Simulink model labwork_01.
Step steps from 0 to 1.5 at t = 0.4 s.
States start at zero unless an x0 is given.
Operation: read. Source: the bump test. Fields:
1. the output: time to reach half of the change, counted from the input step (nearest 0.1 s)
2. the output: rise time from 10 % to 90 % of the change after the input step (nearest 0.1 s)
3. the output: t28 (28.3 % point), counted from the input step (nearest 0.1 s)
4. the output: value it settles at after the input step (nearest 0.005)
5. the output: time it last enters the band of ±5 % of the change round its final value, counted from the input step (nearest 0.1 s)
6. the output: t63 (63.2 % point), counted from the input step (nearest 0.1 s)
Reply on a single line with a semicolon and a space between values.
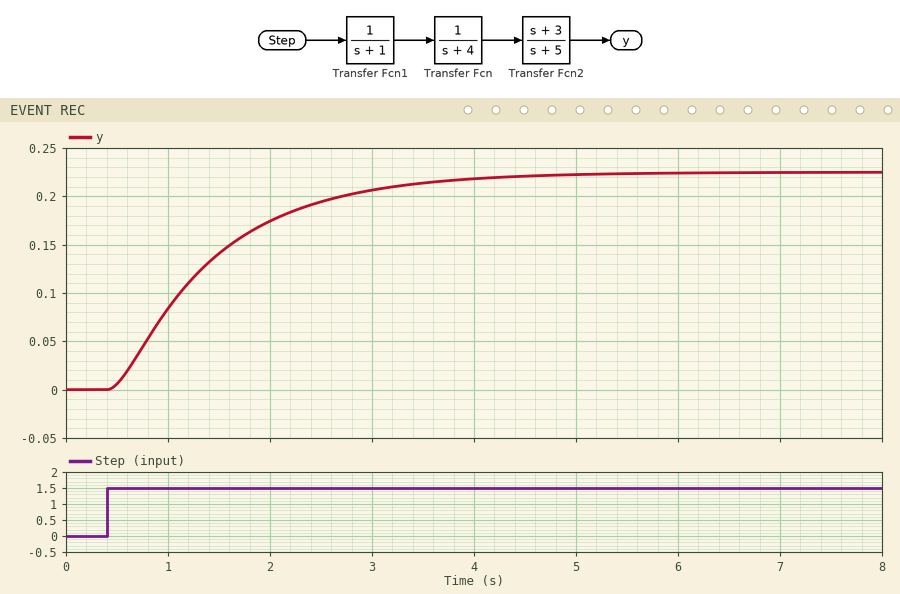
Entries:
0.8 s; 2.2 s; 0.5 s; 0.225; 3.1 s; 1.1 s
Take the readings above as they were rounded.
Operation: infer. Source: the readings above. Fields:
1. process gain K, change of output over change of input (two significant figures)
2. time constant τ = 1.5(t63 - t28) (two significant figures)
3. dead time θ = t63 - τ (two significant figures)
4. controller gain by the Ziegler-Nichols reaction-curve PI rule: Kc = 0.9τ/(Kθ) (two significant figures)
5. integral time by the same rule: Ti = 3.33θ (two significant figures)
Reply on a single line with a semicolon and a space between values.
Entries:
0.15; 0.90 s; 0.20 s; 27; 0.67 s
